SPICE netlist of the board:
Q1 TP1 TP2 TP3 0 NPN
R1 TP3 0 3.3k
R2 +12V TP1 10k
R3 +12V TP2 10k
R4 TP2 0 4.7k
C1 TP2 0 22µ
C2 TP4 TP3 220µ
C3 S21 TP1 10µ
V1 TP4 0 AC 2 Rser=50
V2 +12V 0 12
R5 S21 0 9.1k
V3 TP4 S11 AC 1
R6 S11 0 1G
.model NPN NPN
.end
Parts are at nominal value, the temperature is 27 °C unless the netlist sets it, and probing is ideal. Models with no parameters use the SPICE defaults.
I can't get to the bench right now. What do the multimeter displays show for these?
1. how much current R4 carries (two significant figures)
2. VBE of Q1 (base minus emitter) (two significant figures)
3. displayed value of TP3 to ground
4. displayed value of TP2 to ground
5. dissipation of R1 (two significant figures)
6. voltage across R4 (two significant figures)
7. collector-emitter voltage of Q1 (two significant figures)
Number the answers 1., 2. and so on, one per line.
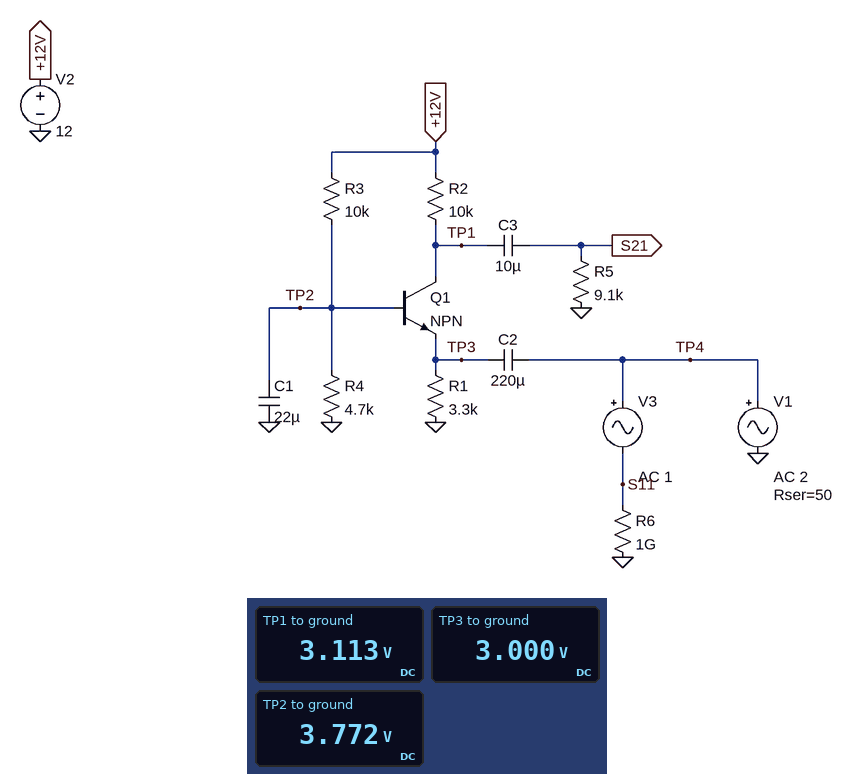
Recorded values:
1. 800 µA
2. 770 mV
3. 3.000 V
4. 3.772 V
5. 2.7 mW
6. 3.8 V
7. 110 mV
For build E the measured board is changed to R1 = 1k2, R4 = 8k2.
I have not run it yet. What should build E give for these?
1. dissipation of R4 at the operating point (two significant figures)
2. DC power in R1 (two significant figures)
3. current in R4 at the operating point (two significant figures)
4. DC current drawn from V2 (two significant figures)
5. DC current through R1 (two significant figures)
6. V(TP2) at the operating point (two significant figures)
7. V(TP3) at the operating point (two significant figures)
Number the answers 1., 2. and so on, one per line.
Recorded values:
1. 900 µW
2. 3.1 mW
3. 330 µA
4. 1.9 mA
5. 1.6 mA
6. 2.7 V
7. 1.9 V
